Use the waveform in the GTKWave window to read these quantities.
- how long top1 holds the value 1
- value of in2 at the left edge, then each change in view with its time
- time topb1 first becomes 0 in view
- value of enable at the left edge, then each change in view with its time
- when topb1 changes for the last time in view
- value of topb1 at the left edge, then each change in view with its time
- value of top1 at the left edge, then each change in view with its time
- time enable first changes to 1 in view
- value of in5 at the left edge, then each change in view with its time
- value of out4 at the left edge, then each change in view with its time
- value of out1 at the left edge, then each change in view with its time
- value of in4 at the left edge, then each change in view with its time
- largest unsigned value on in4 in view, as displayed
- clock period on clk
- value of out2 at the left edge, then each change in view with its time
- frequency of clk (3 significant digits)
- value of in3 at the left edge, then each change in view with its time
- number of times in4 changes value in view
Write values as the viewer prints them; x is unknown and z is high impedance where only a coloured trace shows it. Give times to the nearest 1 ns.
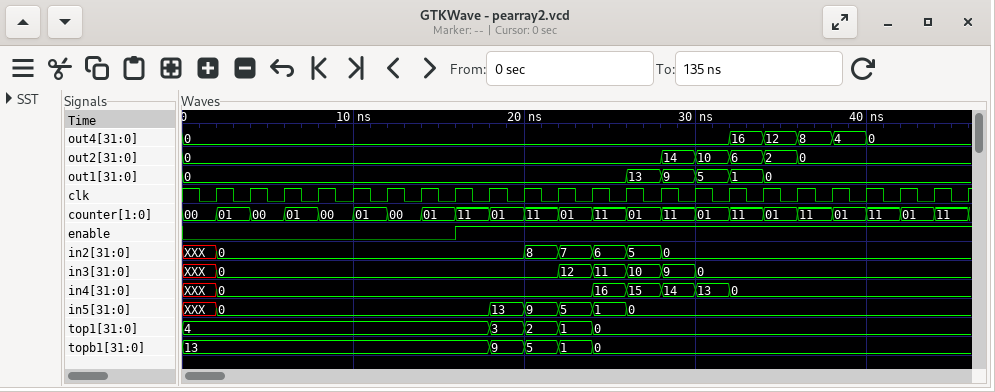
2 ns
XXX, 0 at 2 ns, 8 at 20 ns, 7 at 22 ns, 6 at 24 ns, 5 at 26 ns, 0 at 28 ns
24 ns
0, 1 at 16 ns
24 ns
13, 9 at 18 ns, 5 at 20 ns, 1 at 22 ns, 0 at 24 ns
4, 3 at 18 ns, 2 at 20 ns, 1 at 22 ns, 0 at 24 ns
16 ns
XXX, 0 at 2 ns, 13 at 18 ns, 9 at 20 ns, 5 at 22 ns, 1 at 24 ns, 0 at 26 ns
0, 16 at 32 ns, 12 at 34 ns, 8 at 36 ns, 4 at 38 ns, 0 at 40 ns
0, 13 at 26 ns, 9 at 28 ns, 5 at 30 ns, 1 at 32 ns, 0 at 34 ns
XXX, 0 at 2 ns, 16 at 24 ns, 15 at 26 ns, 14 at 28 ns, 13 at 30 ns, 0 at 32 ns
16
2 ns
0, 14 at 28 ns, 10 at 30 ns, 6 at 32 ns, 2 at 34 ns, 0 at 36 ns
500 MHz
XXX, 0 at 2 ns, 12 at 22 ns, 11 at 24 ns, 10 at 26 ns, 9 at 28 ns, 0 at 30 ns
6
